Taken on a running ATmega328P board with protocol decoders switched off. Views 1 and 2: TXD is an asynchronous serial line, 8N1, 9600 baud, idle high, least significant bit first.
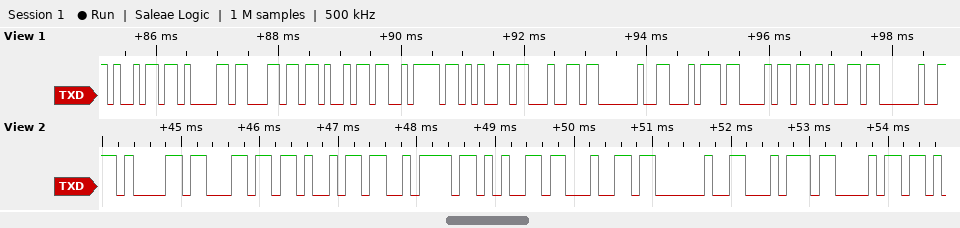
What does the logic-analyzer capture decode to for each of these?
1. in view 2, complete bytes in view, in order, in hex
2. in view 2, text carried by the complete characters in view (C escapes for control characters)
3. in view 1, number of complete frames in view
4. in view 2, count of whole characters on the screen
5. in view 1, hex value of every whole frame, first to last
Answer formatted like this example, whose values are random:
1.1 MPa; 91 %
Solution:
61 6C 69 7A 65 64 20 74 68; "alized th"; 12; 9; 69 61 6C 69 7A 65 64 20 74 68 65 20
